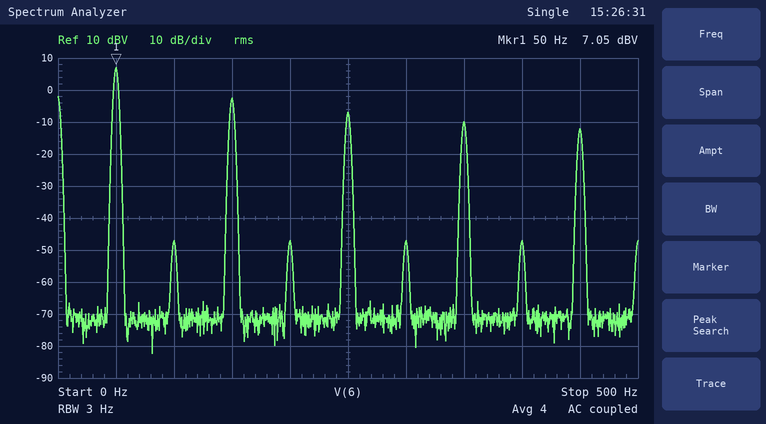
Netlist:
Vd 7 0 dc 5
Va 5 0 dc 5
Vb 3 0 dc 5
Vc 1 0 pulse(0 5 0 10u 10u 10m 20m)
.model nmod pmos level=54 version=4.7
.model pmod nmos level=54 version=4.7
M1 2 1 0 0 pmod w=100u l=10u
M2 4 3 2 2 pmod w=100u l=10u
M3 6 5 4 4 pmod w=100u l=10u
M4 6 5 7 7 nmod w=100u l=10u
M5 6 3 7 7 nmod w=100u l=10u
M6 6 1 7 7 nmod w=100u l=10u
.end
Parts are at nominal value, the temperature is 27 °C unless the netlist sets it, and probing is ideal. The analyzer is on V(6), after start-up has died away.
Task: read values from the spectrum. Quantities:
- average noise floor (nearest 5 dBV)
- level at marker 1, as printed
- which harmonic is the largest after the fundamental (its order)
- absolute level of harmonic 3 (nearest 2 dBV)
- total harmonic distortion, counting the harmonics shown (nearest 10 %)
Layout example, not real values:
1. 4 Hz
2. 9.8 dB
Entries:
1. -70 dBV
2. 7.05 dBV
3. 3
4. -2 dBV
5. 40 %
